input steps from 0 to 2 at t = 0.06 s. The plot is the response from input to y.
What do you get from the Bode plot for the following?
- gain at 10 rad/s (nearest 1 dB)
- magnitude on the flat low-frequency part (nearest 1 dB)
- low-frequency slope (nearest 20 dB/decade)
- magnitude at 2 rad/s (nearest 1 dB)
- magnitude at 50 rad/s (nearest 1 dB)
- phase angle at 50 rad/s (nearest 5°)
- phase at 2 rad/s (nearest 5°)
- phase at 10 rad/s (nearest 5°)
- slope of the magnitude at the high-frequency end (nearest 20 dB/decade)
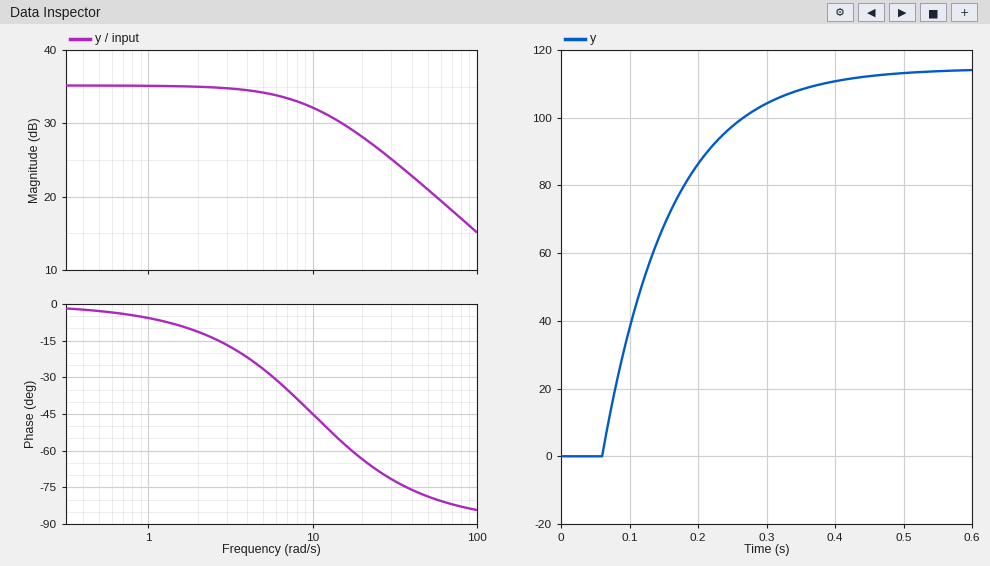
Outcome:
32 dB
35 dB
0 dB/decade
35 dB
21 dB
-80°
-10°
-45°
-20 dB/decade
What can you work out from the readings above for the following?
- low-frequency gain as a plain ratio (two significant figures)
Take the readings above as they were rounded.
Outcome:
56
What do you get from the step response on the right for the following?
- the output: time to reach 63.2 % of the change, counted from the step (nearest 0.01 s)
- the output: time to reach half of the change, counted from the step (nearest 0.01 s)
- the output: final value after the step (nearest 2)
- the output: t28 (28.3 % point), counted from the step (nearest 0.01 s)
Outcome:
0.10 s
0.07 s
114
0.03 s
